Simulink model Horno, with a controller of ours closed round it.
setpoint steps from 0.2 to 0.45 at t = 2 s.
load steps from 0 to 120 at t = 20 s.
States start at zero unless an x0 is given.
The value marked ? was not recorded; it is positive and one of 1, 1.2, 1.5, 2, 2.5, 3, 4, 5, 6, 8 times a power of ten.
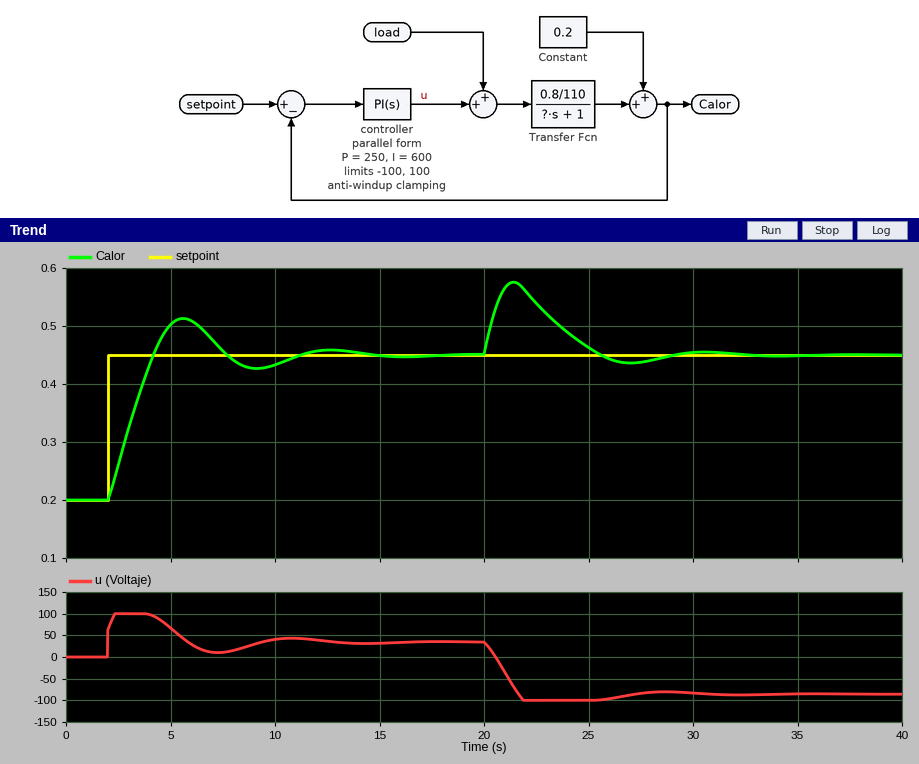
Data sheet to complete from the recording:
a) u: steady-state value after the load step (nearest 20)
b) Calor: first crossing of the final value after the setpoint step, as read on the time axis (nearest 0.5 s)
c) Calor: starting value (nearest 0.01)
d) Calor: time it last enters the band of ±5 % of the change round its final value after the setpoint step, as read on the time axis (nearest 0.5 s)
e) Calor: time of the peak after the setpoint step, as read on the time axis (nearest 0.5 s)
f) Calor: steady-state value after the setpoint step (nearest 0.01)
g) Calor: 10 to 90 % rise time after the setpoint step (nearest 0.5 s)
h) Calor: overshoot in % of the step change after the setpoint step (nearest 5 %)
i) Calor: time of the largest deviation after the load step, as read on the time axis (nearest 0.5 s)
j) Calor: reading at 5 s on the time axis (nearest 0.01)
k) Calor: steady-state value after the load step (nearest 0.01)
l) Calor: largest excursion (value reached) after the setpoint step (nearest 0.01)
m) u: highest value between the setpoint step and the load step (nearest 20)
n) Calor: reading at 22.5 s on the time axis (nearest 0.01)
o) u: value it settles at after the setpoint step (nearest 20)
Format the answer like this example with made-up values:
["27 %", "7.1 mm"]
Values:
["-80", "4.0 s", "0.20", "10.5 s", "5.5 s", "0.45", "1.5 s", "25 %", "21.5 s", "0.50", "0.45", "0.51", "100", "0.54", "40"]
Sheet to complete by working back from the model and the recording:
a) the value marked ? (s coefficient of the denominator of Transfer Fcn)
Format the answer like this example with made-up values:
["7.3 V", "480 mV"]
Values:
["5"]
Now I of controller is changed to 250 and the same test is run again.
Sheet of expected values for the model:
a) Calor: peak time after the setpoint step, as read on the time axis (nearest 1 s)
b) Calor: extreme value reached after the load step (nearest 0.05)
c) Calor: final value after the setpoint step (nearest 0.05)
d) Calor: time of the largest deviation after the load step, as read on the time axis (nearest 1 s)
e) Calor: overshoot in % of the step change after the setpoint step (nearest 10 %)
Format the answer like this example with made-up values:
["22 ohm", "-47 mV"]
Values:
["7 s", "0.60", "0.45", "22 s", "20 %"]
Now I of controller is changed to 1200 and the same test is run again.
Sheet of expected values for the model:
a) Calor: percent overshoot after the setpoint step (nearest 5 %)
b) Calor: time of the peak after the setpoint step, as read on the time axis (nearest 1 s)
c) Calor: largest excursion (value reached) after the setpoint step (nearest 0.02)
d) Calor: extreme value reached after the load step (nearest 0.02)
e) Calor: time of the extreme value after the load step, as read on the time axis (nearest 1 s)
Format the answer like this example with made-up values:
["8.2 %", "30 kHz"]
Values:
["20 %", "5 s", "0.50", "0.54", "21 s"]
